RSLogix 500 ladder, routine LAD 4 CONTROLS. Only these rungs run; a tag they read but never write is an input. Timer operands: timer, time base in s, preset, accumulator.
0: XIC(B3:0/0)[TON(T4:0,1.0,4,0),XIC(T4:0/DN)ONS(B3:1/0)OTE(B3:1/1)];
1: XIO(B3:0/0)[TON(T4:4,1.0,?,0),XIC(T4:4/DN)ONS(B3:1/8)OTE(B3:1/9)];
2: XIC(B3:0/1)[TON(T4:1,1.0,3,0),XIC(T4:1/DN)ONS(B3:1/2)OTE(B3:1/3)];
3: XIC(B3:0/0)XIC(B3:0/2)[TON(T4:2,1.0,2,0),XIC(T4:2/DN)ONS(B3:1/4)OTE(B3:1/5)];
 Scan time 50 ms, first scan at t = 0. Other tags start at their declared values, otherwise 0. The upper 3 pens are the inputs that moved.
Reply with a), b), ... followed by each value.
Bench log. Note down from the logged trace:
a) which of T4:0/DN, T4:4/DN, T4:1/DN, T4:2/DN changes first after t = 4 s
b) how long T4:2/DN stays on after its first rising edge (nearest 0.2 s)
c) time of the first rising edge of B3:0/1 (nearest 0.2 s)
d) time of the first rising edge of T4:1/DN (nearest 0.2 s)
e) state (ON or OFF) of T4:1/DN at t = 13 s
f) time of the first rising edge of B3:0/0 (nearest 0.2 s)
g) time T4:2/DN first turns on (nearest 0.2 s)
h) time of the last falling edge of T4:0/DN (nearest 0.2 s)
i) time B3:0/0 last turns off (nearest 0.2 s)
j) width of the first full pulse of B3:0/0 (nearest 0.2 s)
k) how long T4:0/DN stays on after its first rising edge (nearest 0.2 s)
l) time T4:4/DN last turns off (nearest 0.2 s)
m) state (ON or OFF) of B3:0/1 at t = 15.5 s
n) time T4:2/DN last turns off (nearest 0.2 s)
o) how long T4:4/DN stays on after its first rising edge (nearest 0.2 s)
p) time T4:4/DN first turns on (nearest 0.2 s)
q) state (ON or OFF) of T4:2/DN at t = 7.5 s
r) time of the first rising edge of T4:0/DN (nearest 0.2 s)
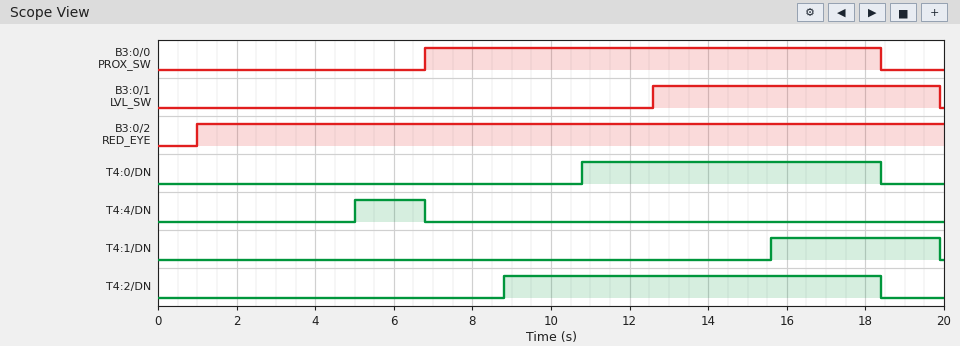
a) T4:4/DN
b) 9.6 s
c) 12.6 s
d) 15.6 s
e) OFF
f) 6.8 s
g) 8.8 s
h) 18.4 s
i) 18.4 s
j) 11.6 s
k) 7.6 s
l) 6.8 s
m) ON
n) 18.4 s
o) 1.8 s
p) 5.0 s
q) OFF
r) 10.8 s
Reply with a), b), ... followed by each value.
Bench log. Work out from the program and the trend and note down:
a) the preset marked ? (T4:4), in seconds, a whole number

a) 5 s
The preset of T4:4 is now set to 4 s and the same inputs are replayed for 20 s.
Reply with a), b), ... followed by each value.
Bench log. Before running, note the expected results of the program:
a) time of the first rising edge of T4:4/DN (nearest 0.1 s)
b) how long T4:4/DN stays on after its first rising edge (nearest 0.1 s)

a) 4.0 s
b) 2.8 s
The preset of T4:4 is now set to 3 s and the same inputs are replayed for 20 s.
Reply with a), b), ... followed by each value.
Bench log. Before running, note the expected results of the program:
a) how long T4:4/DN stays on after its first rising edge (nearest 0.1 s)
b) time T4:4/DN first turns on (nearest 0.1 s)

a) 3.8 s
b) 3.0 s
